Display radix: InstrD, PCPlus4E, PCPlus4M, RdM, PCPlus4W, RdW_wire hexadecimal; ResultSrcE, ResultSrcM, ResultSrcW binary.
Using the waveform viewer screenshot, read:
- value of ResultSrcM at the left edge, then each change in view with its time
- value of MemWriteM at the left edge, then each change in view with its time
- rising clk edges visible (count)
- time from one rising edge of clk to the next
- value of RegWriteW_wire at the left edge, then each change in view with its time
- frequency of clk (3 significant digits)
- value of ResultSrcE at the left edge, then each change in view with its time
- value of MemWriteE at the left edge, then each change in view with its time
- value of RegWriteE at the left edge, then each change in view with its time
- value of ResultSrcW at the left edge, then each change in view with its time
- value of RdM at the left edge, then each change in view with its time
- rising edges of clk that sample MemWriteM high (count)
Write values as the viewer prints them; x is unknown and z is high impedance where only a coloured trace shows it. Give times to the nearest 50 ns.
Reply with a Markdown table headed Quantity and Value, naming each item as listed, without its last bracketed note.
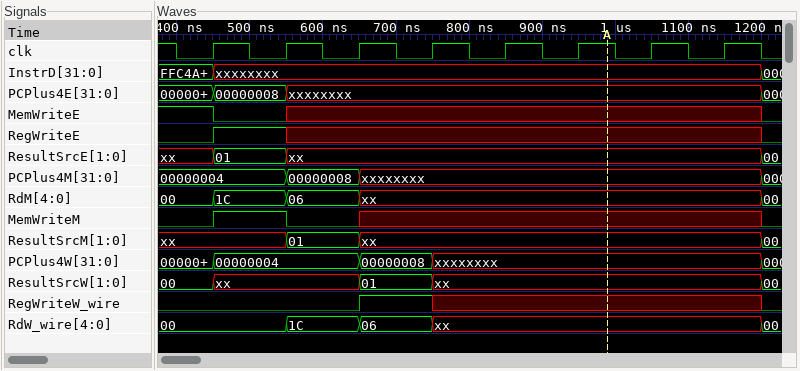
| Quantity | Value |
|---|---|
| value of ResultSrcM at the left edge, then each change in view with its time | xx, 01 at 550 ns, xx at 650 ns, 00 at 1200 ns |
| value of MemWriteM at the left edge, then each change in view with its time | 0, 1 at 450 ns, 0 at 550 ns, x at 650 ns, 0 at 1200 ns |
| rising clk edges visible | 8 |
| time from one rising edge of clk to the next | 100 ns |
| value of RegWriteW_wire at the left edge, then each change in view with its time | 0, 1 at 650 ns, x at 750 ns, 0 at 1200 ns |
| frequency of clk | 10.0 MHz |
| value of ResultSrcE at the left edge, then each change in view with its time | xx, 01 at 450 ns, xx at 550 ns, 00 at 1200 ns |
| value of MemWriteE at the left edge, then each change in view with its time | 1, 0 at 450 ns, x at 550 ns, 0 at 1200 ns |
| value of RegWriteE at the left edge, then each change in view with its time | 0, 1 at 450 ns, x at 550 ns, 0 at 1200 ns |
| value of ResultSrcW at the left edge, then each change in view with its time | 00, xx at 450 ns, 01 at 650 ns, xx at 750 ns, 00 at 1200 ns |
| value of RdM at the left edge, then each change in view with its time | 00, 1C at 450 ns, 06 at 550 ns, xx at 650 ns, 00 at 1200 ns |
| rising edges of clk that sample MemWriteM high | 1 |
